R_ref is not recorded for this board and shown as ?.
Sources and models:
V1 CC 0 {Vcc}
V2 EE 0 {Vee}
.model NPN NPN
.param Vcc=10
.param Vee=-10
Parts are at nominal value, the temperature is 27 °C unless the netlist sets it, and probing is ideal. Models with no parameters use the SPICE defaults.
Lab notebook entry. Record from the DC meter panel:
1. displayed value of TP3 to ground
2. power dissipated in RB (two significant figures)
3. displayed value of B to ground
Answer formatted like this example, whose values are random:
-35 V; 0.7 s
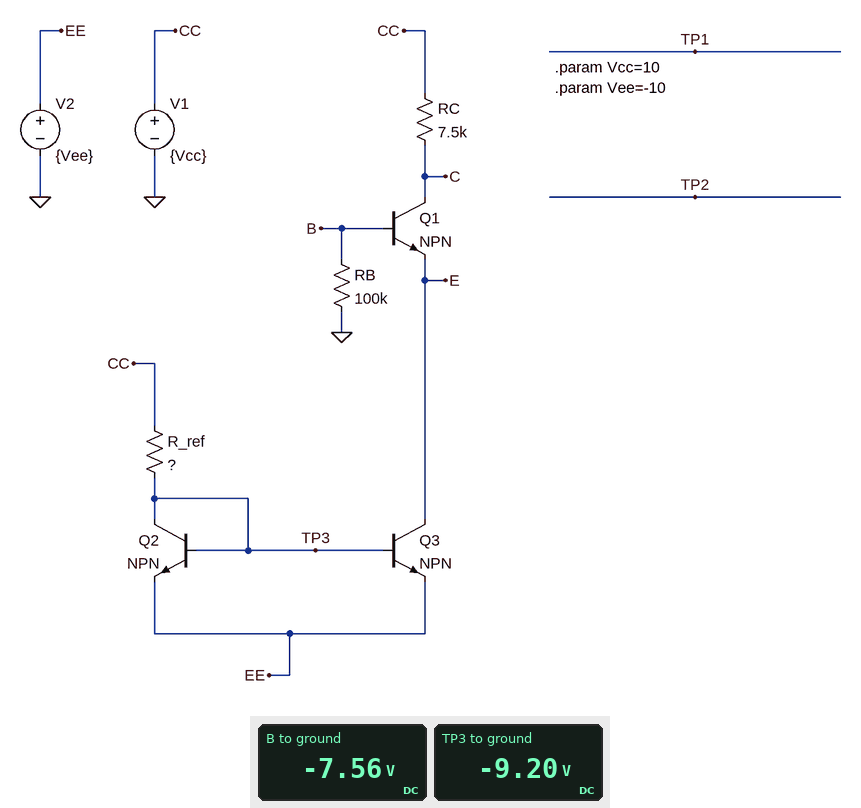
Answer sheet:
-9.20 V; 570 µW; -7.56 V
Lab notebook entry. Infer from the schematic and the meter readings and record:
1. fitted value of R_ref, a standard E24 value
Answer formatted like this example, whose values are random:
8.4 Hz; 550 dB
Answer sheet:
7.5 kΩ
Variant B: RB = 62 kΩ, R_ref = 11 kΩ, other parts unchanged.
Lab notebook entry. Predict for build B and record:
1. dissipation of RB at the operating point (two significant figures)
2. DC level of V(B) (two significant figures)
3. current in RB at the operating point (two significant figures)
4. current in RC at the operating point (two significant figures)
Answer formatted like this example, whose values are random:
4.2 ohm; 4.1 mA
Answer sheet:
61 µW; -1.9 V; 31 µA; 1.7 mA
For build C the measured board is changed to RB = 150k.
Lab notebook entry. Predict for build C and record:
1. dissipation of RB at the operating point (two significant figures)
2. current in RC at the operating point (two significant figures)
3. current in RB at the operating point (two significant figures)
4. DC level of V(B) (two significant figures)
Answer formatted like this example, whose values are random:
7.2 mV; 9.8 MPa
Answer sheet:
400 µW; 2.5 mA; 52 µA; -7.8 V
